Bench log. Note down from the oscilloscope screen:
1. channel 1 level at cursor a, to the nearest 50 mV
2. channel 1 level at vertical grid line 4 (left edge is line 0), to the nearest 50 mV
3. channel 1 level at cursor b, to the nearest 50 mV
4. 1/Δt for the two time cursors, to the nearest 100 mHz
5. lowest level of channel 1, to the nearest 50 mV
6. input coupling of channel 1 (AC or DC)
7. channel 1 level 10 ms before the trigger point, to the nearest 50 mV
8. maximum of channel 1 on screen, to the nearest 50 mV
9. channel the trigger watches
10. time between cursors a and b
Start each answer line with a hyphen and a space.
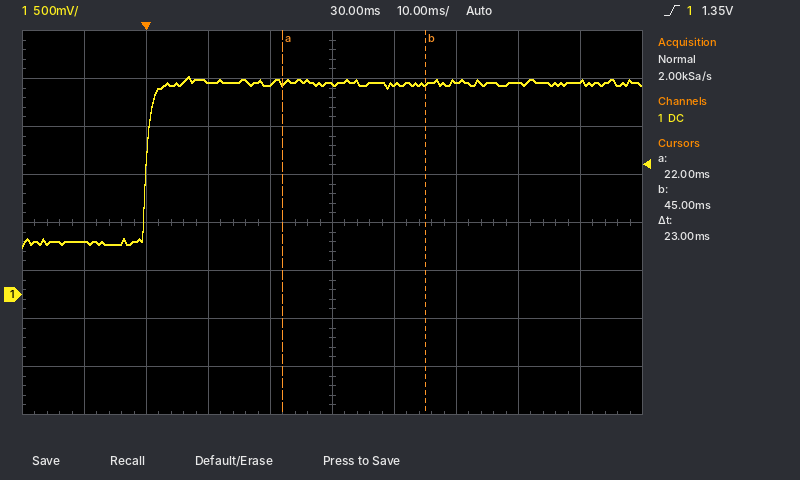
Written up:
- 2.20 V
- 2.20 V
- 2.20 V
- 43.5 Hz
- 500 mV
- DC
- 550 mV
- 2.25 V
- channel 1
- 23 ms
